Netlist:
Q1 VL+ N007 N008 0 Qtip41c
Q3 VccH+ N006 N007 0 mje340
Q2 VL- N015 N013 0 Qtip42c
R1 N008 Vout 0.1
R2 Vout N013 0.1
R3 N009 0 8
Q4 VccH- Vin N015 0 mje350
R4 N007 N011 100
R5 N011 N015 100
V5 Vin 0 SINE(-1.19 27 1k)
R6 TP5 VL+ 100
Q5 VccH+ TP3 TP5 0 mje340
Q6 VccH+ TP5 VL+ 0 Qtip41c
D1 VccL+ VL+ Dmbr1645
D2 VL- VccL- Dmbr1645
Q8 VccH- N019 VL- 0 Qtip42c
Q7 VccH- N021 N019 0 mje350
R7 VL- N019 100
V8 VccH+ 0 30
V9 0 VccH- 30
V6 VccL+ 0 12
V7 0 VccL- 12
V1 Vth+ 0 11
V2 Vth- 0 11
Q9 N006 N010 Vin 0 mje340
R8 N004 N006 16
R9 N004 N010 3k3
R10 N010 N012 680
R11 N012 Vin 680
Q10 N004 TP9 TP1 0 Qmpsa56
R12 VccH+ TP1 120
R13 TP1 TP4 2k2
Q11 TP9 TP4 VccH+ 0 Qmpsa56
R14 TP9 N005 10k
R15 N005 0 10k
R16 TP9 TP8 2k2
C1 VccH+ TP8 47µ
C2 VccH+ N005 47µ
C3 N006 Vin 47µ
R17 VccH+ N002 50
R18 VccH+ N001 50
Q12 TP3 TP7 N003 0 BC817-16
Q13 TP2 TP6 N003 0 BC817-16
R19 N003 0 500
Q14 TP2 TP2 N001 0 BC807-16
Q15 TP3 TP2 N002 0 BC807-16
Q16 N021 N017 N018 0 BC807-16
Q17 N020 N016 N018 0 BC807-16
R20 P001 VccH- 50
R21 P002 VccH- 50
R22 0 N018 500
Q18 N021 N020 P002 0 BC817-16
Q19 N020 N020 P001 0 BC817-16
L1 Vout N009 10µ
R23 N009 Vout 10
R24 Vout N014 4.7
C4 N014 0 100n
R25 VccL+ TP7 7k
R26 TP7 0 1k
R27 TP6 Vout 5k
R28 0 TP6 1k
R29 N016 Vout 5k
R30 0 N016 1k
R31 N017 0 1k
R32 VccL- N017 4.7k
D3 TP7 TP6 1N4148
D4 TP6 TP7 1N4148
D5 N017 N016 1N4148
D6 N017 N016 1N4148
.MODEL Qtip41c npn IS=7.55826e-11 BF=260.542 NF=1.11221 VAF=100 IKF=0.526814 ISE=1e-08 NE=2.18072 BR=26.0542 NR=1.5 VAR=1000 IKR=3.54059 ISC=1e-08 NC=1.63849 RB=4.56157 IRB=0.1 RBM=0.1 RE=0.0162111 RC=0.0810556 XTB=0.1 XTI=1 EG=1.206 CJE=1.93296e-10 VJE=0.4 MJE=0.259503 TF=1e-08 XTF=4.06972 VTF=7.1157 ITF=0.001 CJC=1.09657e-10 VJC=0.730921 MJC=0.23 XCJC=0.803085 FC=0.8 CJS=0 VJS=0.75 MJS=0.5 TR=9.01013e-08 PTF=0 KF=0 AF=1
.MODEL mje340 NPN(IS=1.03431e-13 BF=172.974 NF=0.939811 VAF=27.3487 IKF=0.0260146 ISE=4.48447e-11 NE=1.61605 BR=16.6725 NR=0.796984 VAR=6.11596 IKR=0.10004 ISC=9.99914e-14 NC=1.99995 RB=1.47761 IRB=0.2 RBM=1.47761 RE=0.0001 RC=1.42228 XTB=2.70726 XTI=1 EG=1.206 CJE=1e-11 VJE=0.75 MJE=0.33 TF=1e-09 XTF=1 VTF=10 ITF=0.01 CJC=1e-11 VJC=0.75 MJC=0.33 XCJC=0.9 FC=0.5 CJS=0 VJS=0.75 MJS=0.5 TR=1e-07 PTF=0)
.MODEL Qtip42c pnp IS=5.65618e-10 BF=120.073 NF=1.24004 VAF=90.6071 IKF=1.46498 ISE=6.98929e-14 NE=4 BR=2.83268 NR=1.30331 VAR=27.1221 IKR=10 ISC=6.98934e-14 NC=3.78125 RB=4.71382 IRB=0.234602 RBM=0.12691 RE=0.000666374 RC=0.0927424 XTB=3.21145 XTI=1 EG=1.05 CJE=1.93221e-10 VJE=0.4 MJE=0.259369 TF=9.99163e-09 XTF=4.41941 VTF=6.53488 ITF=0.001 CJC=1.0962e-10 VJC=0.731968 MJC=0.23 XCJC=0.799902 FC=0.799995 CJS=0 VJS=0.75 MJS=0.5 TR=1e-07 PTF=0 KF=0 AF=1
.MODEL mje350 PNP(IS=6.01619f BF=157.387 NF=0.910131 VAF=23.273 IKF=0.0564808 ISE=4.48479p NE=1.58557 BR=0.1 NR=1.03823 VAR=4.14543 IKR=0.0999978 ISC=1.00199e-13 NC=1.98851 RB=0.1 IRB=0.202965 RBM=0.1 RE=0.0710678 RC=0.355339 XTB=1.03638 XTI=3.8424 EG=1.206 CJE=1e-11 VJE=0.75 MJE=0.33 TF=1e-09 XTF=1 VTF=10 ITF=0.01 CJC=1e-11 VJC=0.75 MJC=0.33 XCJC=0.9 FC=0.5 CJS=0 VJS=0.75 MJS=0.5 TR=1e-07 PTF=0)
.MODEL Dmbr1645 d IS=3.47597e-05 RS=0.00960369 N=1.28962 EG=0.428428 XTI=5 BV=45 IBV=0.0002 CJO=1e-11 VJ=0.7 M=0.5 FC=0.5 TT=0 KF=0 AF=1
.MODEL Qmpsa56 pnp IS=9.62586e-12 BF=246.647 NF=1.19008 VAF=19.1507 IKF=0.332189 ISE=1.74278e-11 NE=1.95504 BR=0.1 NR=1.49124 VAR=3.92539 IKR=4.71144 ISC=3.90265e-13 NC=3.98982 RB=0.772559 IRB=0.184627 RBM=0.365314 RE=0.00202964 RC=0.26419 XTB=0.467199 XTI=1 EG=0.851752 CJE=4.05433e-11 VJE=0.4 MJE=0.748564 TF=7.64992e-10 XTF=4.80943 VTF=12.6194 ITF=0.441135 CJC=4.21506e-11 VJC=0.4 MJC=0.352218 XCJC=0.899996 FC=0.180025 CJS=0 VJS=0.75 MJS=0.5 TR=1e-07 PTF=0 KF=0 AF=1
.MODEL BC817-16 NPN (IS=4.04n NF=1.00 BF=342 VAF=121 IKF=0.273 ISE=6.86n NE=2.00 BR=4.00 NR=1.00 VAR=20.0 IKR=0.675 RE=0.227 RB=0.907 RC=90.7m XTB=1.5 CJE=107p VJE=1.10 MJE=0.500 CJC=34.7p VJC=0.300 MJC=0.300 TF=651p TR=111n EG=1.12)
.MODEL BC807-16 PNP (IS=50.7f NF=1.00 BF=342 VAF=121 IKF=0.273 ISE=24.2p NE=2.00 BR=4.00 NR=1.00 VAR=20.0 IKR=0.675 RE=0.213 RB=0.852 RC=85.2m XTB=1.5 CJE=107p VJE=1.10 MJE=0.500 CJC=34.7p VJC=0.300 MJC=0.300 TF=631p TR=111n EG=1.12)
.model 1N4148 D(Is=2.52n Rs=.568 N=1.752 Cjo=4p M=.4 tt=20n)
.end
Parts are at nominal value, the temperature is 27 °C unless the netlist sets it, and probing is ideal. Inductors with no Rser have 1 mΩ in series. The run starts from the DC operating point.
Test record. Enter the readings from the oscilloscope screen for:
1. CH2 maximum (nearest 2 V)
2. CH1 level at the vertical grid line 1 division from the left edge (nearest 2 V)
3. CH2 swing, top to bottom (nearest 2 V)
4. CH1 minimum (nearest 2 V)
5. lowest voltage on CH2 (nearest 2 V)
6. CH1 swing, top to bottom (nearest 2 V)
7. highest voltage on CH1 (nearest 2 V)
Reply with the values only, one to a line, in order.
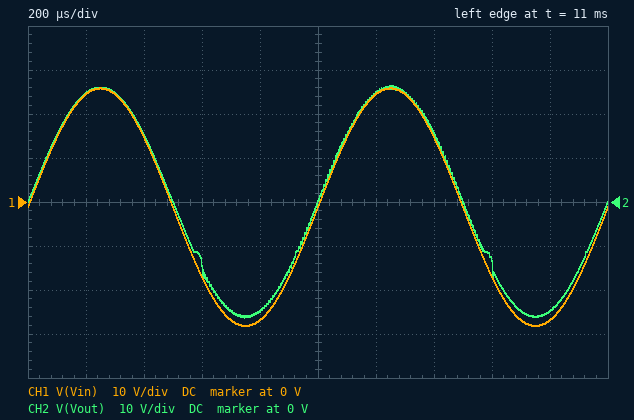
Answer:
26 V
24 V
52 V
-28 V
-26 V
54 V
26 V
